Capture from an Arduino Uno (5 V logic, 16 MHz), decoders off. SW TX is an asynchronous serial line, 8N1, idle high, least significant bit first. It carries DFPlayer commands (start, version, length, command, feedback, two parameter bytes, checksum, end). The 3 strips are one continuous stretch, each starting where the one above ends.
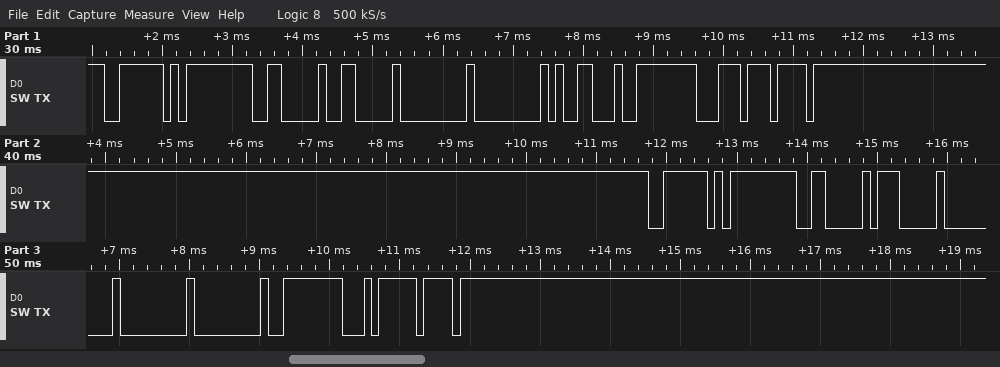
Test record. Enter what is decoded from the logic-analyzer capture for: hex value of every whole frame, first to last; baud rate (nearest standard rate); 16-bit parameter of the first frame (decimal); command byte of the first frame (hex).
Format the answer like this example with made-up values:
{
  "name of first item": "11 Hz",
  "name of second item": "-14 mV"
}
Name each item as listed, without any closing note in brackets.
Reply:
{
  "hex value of every whole frame, first to last": "0x7E 0xFF 0x06 0x06 0x00 0x00 0x19 0xFE 0xDC 0xEF 0x7E 0xFF 0x06 0x07 0x00 0x00 0x00 0xFE 0xF4 0xEF",
  "baud rate": "9600 baud",
  "16-bit parameter of the first frame": "25",
  "command byte of the first frame": "0x06"
}
